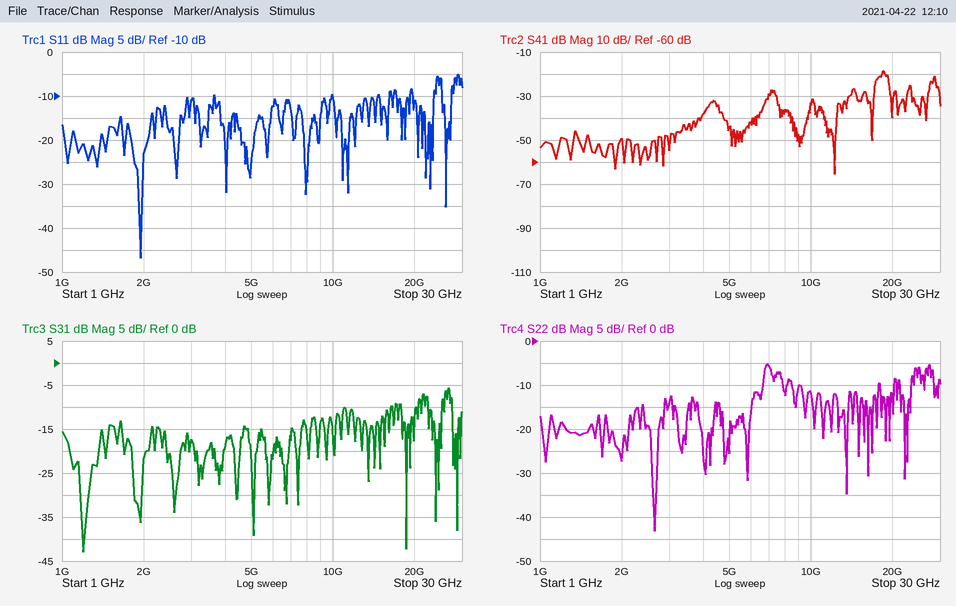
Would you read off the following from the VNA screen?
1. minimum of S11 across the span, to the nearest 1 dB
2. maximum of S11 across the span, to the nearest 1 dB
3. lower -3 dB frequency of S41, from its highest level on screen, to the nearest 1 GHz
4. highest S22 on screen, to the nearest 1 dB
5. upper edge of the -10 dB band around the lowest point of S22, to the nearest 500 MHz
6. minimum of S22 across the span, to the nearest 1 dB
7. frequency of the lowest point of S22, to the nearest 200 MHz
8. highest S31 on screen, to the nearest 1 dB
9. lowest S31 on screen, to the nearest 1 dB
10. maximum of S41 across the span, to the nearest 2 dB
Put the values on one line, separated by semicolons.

-47 dB; -5 dB; 18 GHz; -5 dB; 6.5 GHz; -43 dB; 2.6 GHz; -6 dB; -43 dB; -18 dB
